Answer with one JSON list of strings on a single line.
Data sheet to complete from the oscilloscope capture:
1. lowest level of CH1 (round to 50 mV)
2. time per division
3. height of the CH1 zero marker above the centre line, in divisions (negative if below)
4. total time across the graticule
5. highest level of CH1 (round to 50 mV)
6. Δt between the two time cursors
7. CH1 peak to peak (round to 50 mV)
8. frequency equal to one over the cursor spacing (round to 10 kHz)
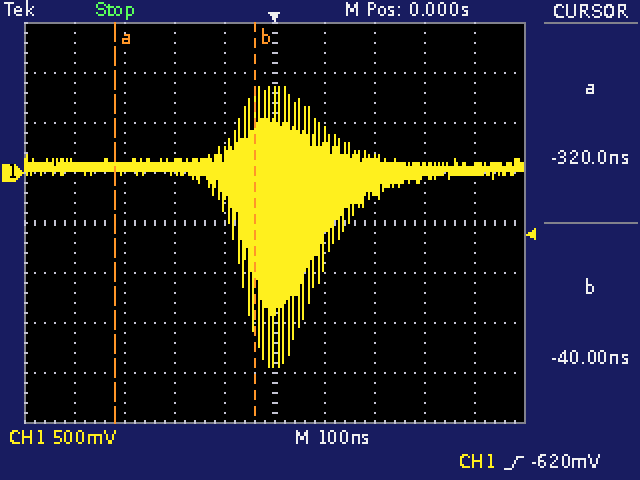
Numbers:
["-1.95 V", "100 ns", "+1.0 div", "1 µs", "850 mV", "280 ns", "2.80 V", "3.57 MHz"]
